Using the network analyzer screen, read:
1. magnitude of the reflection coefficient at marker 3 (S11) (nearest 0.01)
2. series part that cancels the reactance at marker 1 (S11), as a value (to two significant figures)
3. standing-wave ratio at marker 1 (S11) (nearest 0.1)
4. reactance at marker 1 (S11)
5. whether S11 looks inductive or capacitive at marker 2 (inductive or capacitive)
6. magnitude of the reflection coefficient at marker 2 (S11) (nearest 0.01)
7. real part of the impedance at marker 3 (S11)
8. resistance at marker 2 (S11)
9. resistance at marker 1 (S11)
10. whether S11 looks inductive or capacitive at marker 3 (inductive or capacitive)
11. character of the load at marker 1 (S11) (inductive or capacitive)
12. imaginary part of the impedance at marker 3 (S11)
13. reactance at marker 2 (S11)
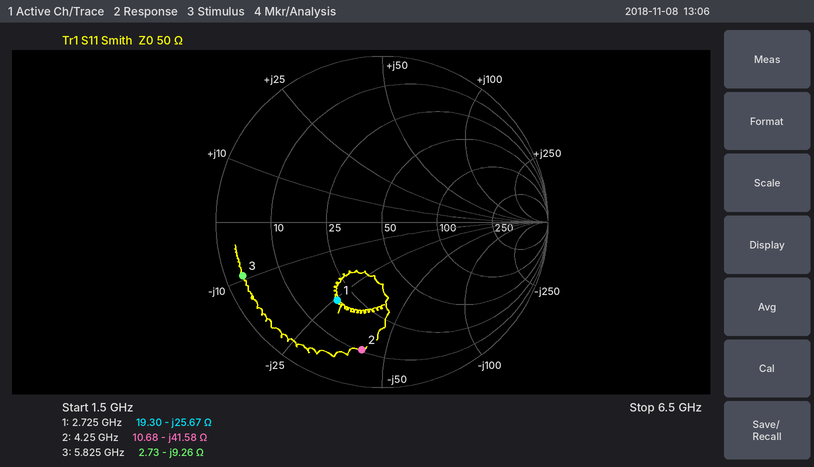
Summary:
0.90
1.5 nH
3.4
-25.67 Ω
capacitive
0.78
2.73 Ω
10.68 Ω
19.30 Ω
capacitive
capacitive
-9.26 Ω
-41.58 Ω
